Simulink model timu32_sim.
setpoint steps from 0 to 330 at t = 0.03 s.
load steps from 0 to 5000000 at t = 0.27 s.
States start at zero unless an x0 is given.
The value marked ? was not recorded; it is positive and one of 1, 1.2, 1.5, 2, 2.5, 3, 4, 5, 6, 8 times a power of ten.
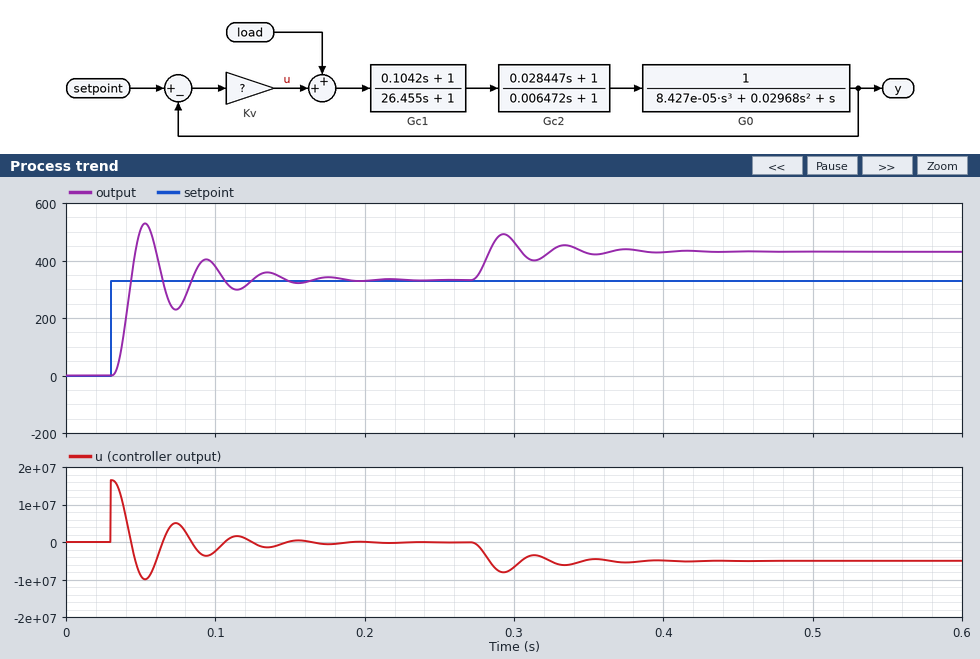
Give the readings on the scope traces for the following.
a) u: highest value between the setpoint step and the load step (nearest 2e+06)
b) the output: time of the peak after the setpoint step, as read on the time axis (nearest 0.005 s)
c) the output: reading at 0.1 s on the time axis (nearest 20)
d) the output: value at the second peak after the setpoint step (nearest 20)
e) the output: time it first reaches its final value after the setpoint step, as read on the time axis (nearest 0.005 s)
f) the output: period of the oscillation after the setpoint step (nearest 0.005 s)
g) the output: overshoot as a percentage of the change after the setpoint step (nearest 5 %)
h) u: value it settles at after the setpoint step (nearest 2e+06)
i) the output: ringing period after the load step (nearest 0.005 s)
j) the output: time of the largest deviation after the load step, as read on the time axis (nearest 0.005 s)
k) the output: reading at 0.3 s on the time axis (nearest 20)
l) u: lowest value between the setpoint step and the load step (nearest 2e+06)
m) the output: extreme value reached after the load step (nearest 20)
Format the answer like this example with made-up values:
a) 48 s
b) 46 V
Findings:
a) 16000000
b) 0.055 s
c) 380
d) 400
e) 0.045 s
f) 0.040 s
g) 60 %
h) 0
i) 0.040 s
j) 0.295 s
k) 460
l) -10000000
m) 500
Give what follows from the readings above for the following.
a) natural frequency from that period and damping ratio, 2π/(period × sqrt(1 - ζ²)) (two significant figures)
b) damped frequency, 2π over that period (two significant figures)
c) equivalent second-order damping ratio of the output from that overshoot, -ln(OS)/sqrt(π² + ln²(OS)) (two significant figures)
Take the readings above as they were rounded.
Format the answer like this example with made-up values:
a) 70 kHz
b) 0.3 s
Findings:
a) 160 rad/s
b) 160 rad/s
c) 0.16
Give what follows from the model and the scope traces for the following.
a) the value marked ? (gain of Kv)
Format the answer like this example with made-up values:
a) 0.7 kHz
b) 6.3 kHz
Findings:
a) 50000
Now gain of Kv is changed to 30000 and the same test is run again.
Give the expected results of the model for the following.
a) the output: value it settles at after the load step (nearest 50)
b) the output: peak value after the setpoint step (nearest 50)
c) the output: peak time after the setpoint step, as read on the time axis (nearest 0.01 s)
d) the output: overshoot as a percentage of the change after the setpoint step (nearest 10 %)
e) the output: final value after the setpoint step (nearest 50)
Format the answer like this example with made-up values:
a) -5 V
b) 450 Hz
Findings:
a) 500
b) 450
c) 0.06 s
d) 40 %
e) 350
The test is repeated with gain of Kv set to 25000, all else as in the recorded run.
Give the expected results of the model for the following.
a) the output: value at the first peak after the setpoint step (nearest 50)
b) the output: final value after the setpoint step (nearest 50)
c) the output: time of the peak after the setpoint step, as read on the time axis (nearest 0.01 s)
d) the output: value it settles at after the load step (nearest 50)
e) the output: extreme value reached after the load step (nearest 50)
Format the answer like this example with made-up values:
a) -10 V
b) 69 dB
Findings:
a) 450
b) 350
c) 0.06 s
d) 550
e) 600
